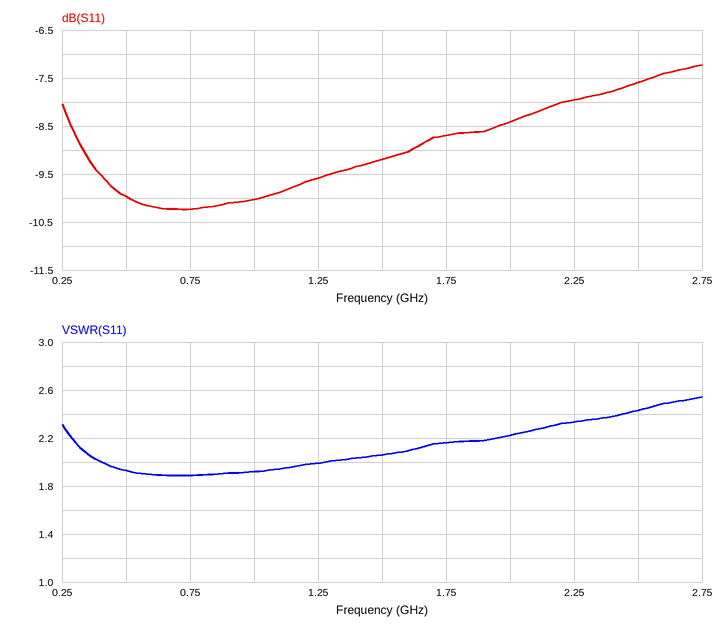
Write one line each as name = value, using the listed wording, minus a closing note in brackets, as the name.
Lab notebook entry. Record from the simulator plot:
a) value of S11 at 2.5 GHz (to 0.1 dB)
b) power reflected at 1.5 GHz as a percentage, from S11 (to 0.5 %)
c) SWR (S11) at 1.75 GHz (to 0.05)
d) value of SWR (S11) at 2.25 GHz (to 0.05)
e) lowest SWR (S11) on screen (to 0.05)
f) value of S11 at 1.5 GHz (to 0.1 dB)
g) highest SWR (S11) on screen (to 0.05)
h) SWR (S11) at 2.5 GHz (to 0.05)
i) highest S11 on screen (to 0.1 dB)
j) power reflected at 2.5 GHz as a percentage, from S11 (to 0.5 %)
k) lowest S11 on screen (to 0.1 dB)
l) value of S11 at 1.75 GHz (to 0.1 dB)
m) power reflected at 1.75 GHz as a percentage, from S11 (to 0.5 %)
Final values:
value of S11 at 2.5 GHz = -7.6 dB
power reflected at 1.5 GHz as a percentage, from S11 = 12.0 %
SWR (S11) at 1.75 GHz = 2.15
value of SWR (S11) at 2.25 GHz = 2.35
lowest SWR (S11) on screen = 1.90
value of S11 at 1.5 GHz = -9.2 dB
highest SWR (S11) on screen = 2.55
SWR (S11) at 2.5 GHz = 2.45
highest S11 on screen = -7.2 dB
power reflected at 2.5 GHz as a percentage, from S11 = 17.5 %
lowest S11 on screen = -10.2 dB
value of S11 at 1.75 GHz = -8.7 dB
power reflected at 1.75 GHz as a percentage, from S11 = 13.5 %
